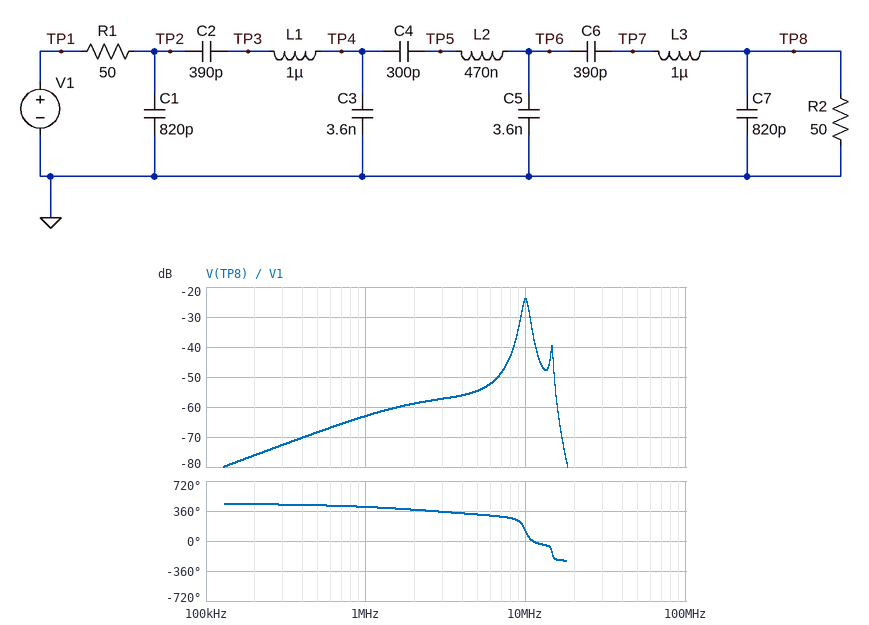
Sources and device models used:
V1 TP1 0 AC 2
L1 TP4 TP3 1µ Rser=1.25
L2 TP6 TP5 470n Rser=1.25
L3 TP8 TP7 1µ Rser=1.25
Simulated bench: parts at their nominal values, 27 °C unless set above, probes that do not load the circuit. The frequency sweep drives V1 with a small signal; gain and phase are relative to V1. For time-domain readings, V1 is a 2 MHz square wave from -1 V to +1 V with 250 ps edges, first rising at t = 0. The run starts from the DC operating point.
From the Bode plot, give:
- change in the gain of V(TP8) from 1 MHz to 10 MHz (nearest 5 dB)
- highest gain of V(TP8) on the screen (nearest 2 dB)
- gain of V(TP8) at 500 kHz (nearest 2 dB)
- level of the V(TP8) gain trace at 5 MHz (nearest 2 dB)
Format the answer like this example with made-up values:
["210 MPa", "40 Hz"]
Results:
["40 dB", "-24 dB", "-68 dB", "-54 dB"]
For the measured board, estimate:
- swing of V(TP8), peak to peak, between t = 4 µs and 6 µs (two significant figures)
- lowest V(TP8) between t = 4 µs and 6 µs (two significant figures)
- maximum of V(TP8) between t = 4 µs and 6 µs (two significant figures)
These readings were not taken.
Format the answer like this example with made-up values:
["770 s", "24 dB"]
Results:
["37 mV", "-19 mV", "19 mV"]
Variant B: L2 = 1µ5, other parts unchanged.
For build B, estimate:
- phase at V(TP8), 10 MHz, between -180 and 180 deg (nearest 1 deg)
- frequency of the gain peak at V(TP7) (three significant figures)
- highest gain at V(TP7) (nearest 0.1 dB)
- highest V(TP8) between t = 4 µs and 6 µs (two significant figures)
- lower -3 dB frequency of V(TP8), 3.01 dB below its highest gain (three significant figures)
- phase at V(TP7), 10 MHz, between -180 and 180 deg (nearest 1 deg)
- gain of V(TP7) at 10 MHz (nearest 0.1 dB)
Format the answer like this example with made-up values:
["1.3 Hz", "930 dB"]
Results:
["-47 deg", "8.01 MHz", "-11.6 dB", "18 mV", "7.90 MHz", "102 deg", "-15.6 dB"]
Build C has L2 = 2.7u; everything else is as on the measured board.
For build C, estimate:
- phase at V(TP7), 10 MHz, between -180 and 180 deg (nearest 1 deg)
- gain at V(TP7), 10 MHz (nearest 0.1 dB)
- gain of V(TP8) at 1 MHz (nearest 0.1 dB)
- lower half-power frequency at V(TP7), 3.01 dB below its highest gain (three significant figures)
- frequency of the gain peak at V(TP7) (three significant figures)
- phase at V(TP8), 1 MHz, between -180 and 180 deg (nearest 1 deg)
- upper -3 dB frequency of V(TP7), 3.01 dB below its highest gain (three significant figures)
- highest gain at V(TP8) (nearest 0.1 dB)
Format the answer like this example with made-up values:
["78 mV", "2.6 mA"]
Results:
["94 deg", "-26.0 dB", "-62.8 dB", "5.94 MHz", "5.99 MHz", "49 deg", "6.04 MHz", "-18.4 dB"]
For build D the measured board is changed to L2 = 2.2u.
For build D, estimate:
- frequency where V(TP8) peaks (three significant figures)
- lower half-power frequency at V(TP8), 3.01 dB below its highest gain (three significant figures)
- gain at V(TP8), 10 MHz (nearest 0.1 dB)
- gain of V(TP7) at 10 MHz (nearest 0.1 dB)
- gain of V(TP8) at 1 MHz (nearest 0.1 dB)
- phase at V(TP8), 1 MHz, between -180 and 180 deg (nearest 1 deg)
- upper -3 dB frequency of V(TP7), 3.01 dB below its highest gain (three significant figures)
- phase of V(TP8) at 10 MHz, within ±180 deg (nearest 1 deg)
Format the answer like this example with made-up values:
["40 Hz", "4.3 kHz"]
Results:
["6.63 MHz", "6.57 MHz", "-31.2 dB", "-23.0 dB", "-62.8 dB", "49 deg", "6.70 MHz", "-54 deg"]
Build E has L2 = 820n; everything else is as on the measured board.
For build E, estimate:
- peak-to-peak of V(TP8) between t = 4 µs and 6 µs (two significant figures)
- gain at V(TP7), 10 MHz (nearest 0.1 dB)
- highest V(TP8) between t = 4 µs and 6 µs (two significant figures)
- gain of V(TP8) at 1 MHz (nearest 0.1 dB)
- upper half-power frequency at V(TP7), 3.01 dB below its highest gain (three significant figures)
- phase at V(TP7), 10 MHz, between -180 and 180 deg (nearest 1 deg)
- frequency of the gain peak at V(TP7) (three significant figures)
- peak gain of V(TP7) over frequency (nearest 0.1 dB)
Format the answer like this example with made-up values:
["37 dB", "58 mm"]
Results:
["89 mV", "-7.3 dB", "44 mV", "-62.9 dB", "11.3 MHz", "-119 deg", "11.1 MHz", "-4.9 dB"]
